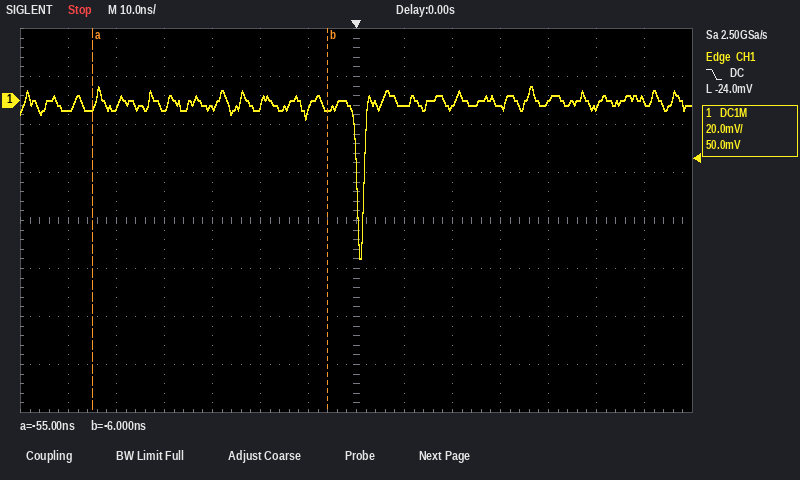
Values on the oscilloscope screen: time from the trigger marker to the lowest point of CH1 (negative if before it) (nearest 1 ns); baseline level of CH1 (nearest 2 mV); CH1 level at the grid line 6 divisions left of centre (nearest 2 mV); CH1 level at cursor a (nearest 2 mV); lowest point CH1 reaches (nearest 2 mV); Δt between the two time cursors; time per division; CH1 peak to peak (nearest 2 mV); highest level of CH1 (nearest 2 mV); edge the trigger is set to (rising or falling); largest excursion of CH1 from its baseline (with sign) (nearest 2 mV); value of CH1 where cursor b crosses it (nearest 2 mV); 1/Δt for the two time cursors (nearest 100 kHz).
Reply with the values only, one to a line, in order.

+1 ns
0 mV
-4 mV
-2 mV
-66 mV
49 ns
10 ns
72 mV
6 mV
falling
-66 mV
-4 mV
20.4 MHz
